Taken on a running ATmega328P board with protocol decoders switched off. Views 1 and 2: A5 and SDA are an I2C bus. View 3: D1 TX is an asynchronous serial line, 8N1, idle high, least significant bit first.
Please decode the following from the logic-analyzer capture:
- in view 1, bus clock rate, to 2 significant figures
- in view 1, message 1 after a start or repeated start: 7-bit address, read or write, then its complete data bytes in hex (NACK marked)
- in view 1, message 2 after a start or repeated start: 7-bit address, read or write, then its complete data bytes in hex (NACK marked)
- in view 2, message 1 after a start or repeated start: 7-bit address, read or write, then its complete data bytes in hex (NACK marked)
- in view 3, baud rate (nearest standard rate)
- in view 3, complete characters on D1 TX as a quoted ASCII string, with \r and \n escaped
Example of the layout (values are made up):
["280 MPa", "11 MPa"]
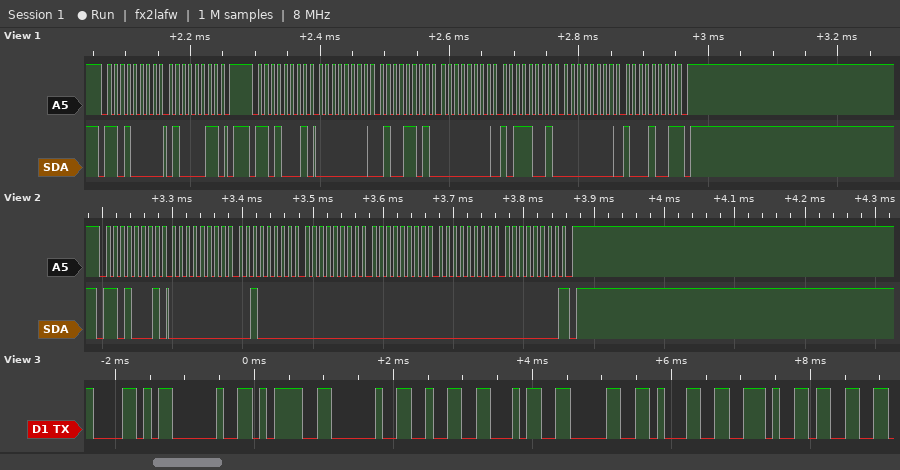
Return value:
["100 kHz", "0x68 write: 43", "0x68 read: 00 4D 00 B9 00 89 NACK", "0x68 read: 00 20 00 00 00 00 NACK", "9600 baud", "\"X = 2401.3\""]
